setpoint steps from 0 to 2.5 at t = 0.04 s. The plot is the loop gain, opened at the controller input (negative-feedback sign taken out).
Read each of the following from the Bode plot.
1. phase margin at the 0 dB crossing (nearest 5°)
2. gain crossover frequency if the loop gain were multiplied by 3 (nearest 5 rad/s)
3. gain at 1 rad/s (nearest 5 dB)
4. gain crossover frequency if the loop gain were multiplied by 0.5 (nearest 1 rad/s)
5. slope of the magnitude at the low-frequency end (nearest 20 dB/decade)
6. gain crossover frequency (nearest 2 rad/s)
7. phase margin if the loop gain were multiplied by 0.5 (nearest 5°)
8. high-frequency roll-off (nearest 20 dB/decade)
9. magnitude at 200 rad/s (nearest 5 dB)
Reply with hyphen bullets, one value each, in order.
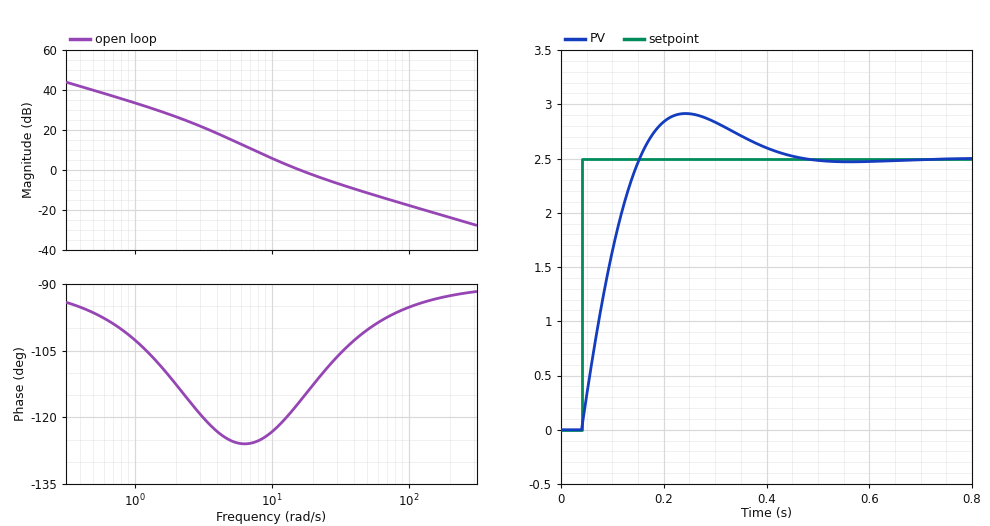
- 65°
- 40 rad/s
- 35 dB
- 10 rad/s
- -20 dB/decade
- 16 rad/s
- 55°
- -20 dB/decade
- -25 dB
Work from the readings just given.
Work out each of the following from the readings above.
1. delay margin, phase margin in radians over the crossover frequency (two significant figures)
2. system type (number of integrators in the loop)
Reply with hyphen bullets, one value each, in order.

- 0.071 s
- 1
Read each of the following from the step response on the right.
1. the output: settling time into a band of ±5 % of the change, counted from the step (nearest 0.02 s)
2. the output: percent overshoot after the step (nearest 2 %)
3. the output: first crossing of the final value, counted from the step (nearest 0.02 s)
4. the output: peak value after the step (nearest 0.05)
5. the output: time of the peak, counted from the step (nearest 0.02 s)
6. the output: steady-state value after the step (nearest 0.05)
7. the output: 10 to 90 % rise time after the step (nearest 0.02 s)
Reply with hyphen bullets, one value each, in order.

- 0.34 s
- 16 %
- 0.12 s
- 2.90
- 0.20 s
- 2.50
- 0.08 s
